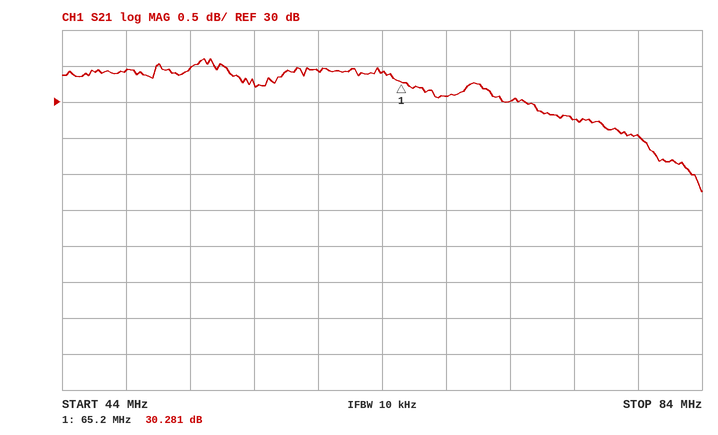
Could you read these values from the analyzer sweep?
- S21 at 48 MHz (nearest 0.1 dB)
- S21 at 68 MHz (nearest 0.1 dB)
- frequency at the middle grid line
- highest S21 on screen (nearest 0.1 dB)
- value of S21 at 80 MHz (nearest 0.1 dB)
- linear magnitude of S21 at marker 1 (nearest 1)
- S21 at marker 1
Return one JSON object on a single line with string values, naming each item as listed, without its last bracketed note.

{"S21 at 48 MHz": "30.4 dB", "S21 at 68 MHz": "30.1 dB", "frequency at the middle grid line": "64 MHz", "highest S21 on screen": "30.6 dB", "value of S21 at 80 MHz": "29.5 dB", "linear magnitude of S21 at marker 1": "33", "S21 at marker 1": "30.281 dB"}
